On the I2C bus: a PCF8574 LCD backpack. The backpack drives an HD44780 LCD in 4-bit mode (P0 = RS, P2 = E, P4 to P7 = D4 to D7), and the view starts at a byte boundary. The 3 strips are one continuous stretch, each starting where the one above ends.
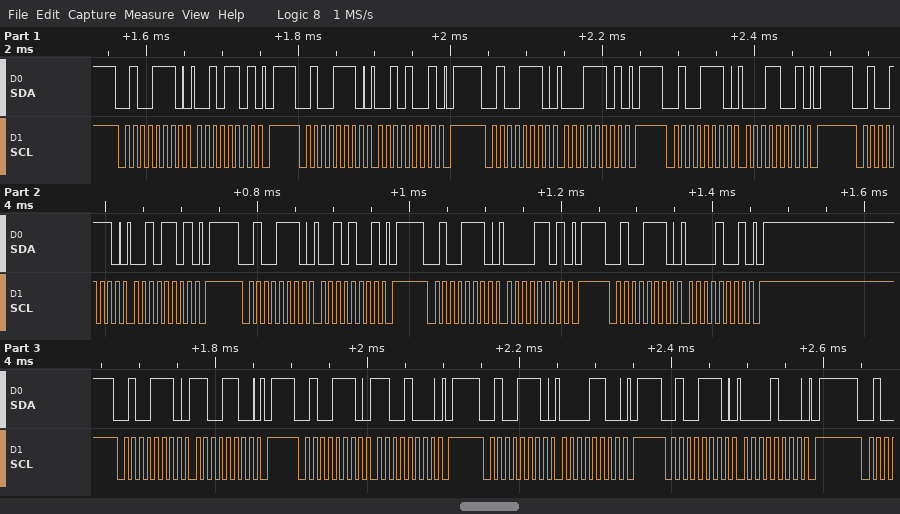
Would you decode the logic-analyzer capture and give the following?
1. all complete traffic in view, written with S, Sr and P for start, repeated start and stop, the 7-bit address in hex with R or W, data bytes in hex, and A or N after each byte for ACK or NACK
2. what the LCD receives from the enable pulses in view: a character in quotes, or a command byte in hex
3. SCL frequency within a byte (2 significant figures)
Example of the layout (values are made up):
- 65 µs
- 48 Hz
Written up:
- S 27W A 2D A P S 27W A 29 A P S 27W A 1D A P S 27W A 19 A P S 27W A 2D A P S 27W A 29 A P S 27W A 0D A P S 27W A 09 A P S 27W A CC A P S 27W A C8 A P S 27W A 0C A P S 27W A 08 A P
- '!' ' ' 0xC0
- 100 kHz
